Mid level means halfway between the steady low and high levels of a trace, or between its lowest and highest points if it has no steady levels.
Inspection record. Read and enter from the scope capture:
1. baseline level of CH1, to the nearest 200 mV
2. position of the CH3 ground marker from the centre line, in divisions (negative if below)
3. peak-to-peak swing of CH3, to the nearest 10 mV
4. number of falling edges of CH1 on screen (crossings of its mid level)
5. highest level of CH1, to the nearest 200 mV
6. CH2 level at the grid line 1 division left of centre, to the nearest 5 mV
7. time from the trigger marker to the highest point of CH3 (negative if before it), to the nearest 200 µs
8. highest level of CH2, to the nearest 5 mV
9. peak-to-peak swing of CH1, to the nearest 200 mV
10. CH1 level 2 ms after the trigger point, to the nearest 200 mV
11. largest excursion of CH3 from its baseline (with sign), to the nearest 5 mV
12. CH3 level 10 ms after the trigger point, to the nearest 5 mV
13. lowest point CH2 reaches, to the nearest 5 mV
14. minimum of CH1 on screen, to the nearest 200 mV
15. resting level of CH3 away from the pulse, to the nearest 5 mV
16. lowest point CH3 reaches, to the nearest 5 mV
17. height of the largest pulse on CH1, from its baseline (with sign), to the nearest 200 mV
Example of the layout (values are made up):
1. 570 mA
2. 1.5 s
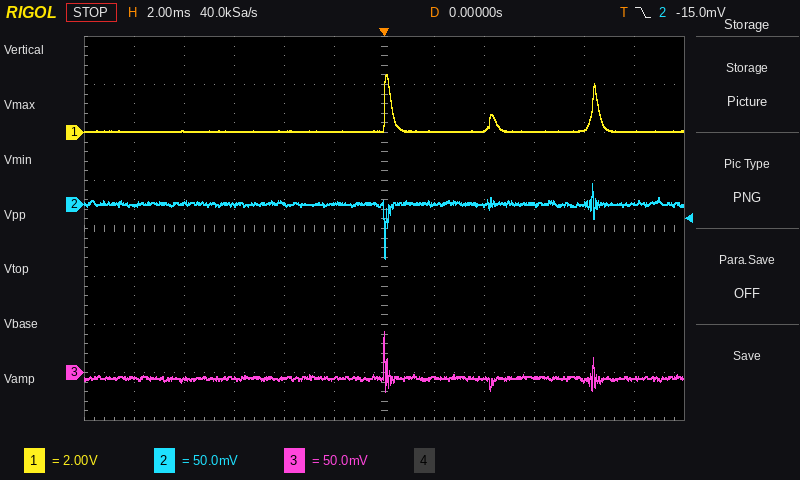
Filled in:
1. 0.0 V
2. -3.0 div
3. 60 mV
4. 2
5. 2.4 V
6. 0 mV
7. 0.0 ms
8. 20 mV
9. 2.4 V
10. 0.0 V
11. +50 mV
12. -5 mV
13. -55 mV
14. 0.0 V
15. -5 mV
16. -20 mV
17. +2.4 V
